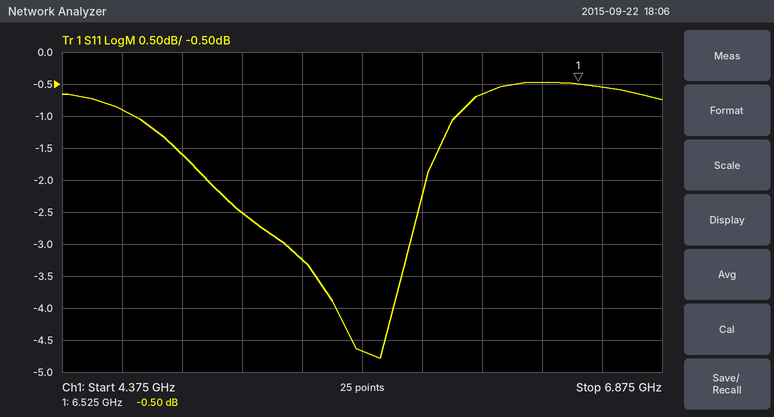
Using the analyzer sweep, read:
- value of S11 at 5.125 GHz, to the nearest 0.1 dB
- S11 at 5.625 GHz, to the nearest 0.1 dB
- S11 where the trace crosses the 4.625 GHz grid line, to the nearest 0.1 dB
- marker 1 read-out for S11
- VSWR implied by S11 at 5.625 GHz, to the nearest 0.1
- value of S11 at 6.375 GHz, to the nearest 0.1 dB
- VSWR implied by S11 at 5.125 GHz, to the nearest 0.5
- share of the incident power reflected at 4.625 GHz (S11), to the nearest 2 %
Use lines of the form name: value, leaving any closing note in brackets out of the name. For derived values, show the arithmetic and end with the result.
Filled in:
value of S11 at 5.125 GHz, to the nearest 0.1 dB: -2.5 dB
S11 at 5.625 GHz, to the nearest 0.1 dB: -4.7 dB
S11 where the trace crosses the 4.625 GHz grid line, to the nearest 0.1 dB: -0.9 dB
marker 1 read-out for S11: -0.50 dB
VSWR implied by S11 at 5.625 GHz, to the nearest 0.1: |Γ| = 10^(-4.7/20) = 0.5821; VSWR = (1 + 0.5821)/(1 − 0.5821) ≈ 3.8
value of S11 at 6.375 GHz, to the nearest 0.1 dB: -0.5 dB
VSWR implied by S11 at 5.125 GHz, to the nearest 0.5: |Γ| = 10^(-2.5/20) = 0.7499; VSWR = (1 + 0.7499)/(1 − 0.7499) ≈ 7.0
share of the incident power reflected at 4.625 GHz (S11), to the nearest 2 %: 10^(-0.9/10) ≈ 81.3 %, so 82 % to the nearest 2 %
